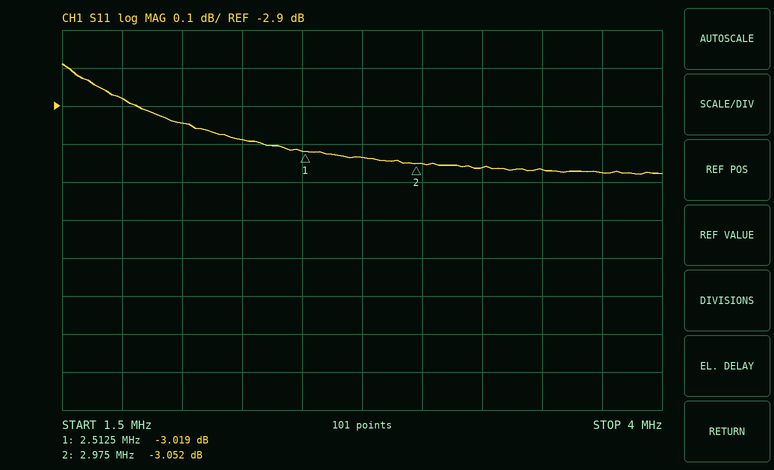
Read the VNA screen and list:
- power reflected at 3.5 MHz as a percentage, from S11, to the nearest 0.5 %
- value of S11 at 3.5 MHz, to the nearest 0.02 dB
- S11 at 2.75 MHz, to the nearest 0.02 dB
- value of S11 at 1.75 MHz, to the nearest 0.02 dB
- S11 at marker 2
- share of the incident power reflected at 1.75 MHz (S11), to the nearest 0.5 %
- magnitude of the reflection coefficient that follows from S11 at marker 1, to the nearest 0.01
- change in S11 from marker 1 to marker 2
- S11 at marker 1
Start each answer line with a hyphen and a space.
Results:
- 49.5 %
- -3.06 dB
- -3.04 dB
- -2.88 dB
- -3.052 dB
- 51.5 %
- 0.71
- -0.033 dB
- -3.019 dB
